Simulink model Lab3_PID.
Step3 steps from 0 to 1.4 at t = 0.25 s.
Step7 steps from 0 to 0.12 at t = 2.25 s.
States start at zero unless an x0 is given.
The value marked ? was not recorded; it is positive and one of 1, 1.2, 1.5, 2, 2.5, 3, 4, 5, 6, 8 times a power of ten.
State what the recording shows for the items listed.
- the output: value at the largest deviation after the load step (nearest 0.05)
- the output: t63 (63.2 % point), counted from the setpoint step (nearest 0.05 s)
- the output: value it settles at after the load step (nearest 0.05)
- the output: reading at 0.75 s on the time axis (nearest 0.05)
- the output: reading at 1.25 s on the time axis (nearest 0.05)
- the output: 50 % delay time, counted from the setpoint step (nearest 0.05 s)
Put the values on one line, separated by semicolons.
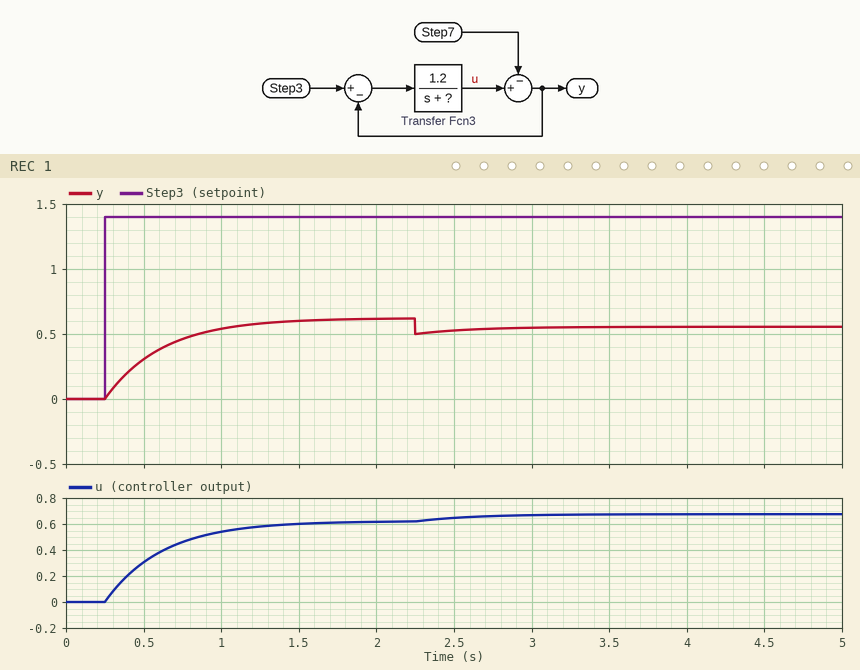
0.50; 0.35 s; 0.55; 0.45; 0.60; 0.25 s
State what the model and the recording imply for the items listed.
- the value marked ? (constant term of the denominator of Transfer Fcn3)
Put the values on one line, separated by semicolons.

1.5
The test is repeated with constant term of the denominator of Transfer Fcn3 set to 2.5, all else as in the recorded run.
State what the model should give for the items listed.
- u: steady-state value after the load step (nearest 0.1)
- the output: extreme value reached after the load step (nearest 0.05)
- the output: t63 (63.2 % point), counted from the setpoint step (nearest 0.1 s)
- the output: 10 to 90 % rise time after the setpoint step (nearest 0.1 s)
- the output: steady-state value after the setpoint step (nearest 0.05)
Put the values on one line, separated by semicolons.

0.5; 0.35; 0.3 s; 0.6 s; 0.45
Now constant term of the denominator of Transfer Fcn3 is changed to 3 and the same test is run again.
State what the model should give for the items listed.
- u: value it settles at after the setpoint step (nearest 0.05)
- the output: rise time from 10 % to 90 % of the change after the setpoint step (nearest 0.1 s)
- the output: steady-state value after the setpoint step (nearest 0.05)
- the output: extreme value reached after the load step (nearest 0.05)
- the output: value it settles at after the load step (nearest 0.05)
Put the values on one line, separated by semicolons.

0.40; 0.5 s; 0.40; 0.30; 0.30
